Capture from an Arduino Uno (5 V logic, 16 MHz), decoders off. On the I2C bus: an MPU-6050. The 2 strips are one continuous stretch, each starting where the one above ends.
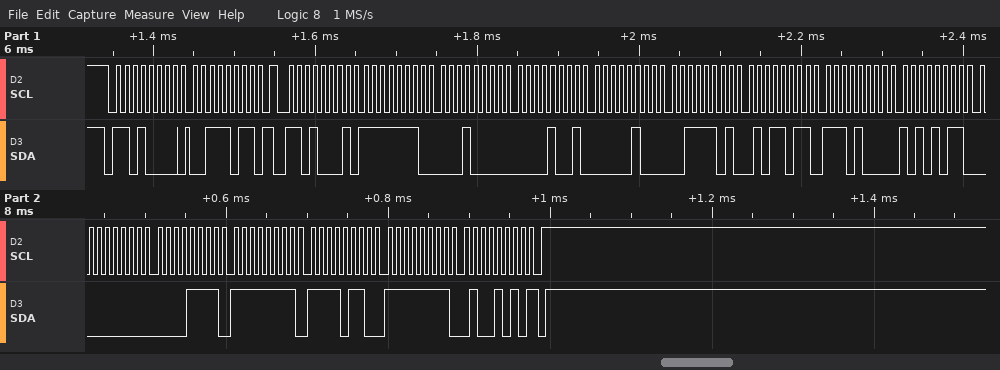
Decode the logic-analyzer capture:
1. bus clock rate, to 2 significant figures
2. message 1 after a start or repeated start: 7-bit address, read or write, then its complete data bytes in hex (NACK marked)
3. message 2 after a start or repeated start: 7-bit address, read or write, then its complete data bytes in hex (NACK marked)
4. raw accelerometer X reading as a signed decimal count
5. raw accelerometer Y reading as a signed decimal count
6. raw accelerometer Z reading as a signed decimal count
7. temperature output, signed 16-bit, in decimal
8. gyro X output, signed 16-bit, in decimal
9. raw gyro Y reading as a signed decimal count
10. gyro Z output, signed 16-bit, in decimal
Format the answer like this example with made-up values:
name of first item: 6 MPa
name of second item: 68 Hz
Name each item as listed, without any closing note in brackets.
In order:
bus clock rate, to 2 significant figures: 100 kHz
message 1 after a start or repeated start: 7-bit address, read or write, then its complete data bytes in hex: 0x68 write: 3B
message 2 after a start or repeated start: 7-bit address, read or write, then its complete data bytes in hex: 0x68 read: FE 10 09 04 3D 5B E8 AB 00 0F FF F6 FF 4A NACK
raw accelerometer X reading as a signed decimal count: -496
raw accelerometer Y reading as a signed decimal count: 2308
raw accelerometer Z reading as a signed decimal count: 15707
temperature output, signed 16-bit, in decimal: -5973
gyro X output, signed 16-bit, in decimal: 15
raw gyro Y reading as a signed decimal count: -10
gyro Z output, signed 16-bit, in decimal: -182
